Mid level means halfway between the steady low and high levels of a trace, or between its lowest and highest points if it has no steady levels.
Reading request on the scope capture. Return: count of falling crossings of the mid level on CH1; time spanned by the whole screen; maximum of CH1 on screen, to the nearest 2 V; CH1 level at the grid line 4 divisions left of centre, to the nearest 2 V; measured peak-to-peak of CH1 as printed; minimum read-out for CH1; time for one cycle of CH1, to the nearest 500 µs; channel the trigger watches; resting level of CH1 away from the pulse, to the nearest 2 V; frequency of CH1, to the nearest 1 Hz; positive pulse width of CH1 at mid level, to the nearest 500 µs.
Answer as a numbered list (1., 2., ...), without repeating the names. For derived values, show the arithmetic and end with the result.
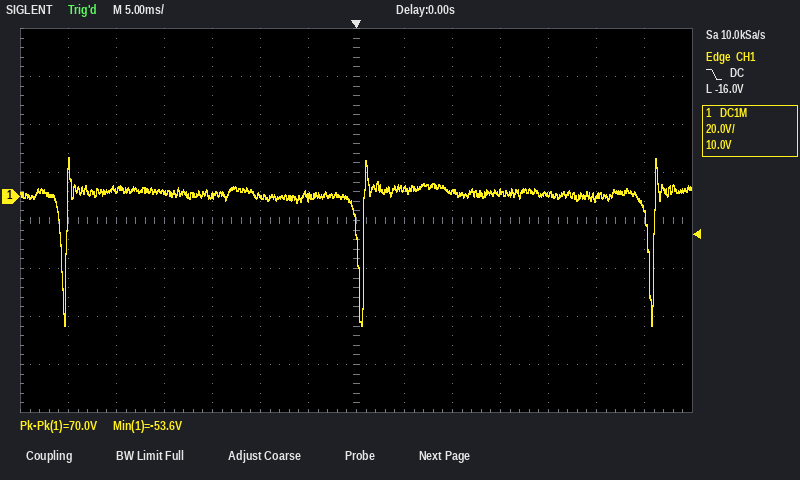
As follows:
1. 3
2. 70 ms
3. 16 V
4. 2 V
5. 70.0 V
6. -53.6 V
7. 30.5 ms
8. CH1
9. 2 V
10. 1 / 30.5 ms ≈ 33 Hz
11. 30.0 ms
